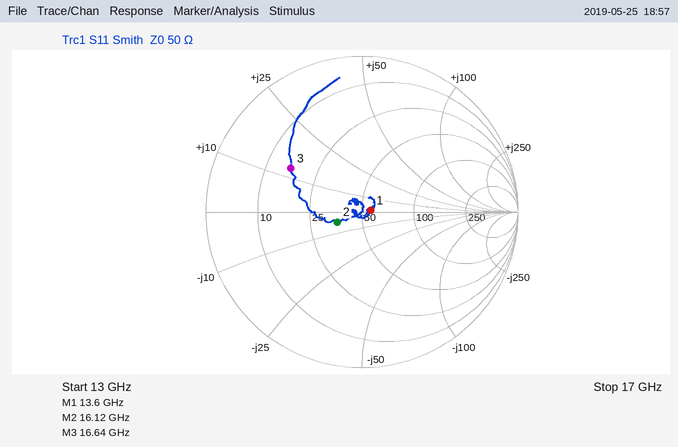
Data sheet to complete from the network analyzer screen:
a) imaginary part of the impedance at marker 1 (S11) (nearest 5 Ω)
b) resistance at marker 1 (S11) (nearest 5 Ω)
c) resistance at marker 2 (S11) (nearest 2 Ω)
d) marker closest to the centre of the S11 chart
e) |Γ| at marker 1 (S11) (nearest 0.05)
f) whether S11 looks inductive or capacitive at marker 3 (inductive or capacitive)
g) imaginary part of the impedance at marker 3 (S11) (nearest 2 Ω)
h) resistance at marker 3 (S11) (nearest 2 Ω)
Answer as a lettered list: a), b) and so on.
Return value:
a) 0 Ω
b) 55 Ω
c) 36 Ω
d) marker 1
e) 0.05
f) inductive
g) +12 Ω
h) 16 Ω
